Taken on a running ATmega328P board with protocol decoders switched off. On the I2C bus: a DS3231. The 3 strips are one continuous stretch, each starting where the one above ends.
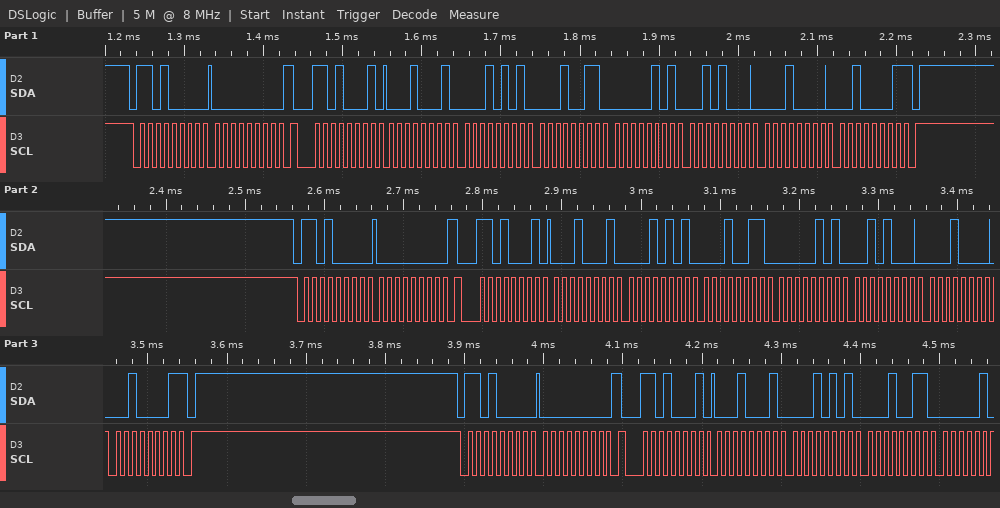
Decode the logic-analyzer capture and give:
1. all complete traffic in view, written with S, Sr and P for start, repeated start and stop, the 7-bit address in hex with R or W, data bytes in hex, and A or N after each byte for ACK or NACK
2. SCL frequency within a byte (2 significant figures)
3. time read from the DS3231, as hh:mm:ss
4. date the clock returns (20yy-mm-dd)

S 68W A 00 A Sr 68R A 11 A 15 A 13 A 05 A 28 A 10 A 21 N P S 68W A 00 A Sr 68R A 11 A 15 A 13 A 05 A 28 A 10 A 21 N P S 68W A 00 A Sr 68R A 11 A 15 A 13 A
100 kHz
13:15:11
2021-10-28
